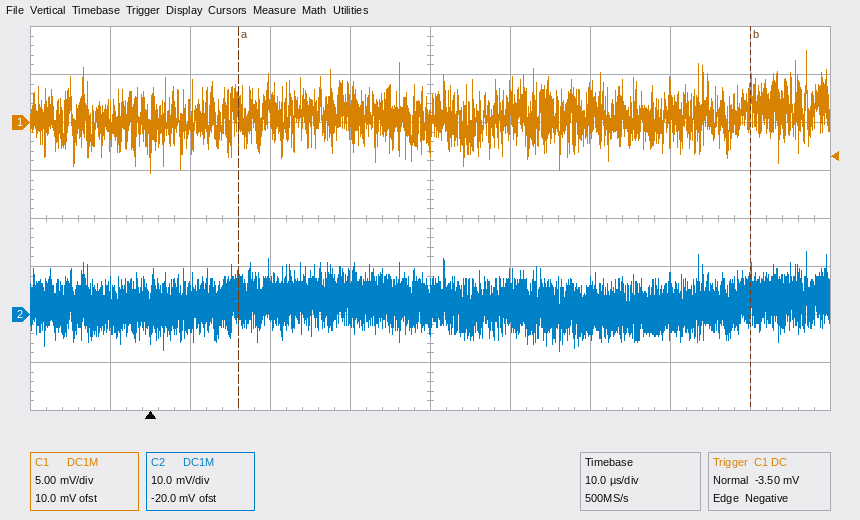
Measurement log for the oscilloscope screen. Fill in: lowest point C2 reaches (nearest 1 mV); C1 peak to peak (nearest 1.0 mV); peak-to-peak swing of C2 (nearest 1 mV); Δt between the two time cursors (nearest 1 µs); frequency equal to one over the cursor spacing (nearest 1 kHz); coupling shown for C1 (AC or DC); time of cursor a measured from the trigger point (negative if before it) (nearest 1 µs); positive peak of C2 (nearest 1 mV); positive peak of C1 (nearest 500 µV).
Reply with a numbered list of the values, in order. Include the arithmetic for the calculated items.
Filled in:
1. -8 mV
2. 13.0 mV
3. 13 mV − (-8 mV) = 21 mV
4. 64 µs
5. 1 / 64 µs ≈ 16 kHz
6. DC
7. +11 µs
8. 13 mV
9. 7.5 mV
